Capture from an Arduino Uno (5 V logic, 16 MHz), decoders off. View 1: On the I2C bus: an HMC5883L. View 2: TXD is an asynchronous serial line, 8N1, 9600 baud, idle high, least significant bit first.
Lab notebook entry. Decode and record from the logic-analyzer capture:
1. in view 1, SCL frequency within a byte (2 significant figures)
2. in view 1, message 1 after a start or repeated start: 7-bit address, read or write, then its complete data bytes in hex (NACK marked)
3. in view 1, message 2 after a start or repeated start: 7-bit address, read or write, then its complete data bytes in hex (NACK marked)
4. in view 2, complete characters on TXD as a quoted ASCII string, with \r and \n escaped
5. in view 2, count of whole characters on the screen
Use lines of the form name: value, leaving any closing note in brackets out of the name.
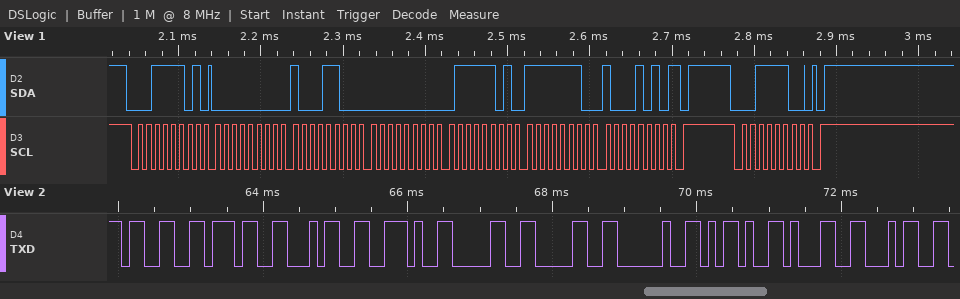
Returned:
in view 1, SCL frequency within a byte: 100 kHz
in view 1, message 1 after a start or repeated start: 7-bit address, read or write, then its complete data bytes in hex: 0x1E read: 00 8C 00 7D FE 8A NACK
in view 1, message 2 after a start or repeated start: 7-bit address, read or write, then its complete data bytes in hex: 0x1E write
in view 2, complete characters on TXD as a quoted ASCII string, with \r and \n escaped: "374.00 -14"
in view 2, count of whole characters on the screen: 10
